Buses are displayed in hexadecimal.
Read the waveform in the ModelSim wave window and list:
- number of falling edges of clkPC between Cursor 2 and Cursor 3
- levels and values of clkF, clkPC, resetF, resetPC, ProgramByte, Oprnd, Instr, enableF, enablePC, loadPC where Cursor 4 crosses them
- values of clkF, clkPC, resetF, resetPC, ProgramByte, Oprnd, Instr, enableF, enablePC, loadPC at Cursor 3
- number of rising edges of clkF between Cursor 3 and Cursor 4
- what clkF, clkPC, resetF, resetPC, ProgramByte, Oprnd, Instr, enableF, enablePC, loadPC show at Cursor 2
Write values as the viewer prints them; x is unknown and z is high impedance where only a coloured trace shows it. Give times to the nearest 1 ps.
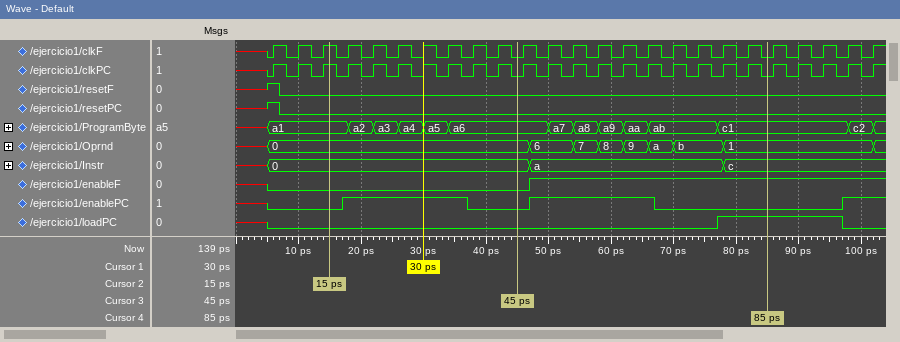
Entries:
8
clkF=0, clkPC=0, resetF=0, resetPC=0, ProgramByte=c1, Oprnd=1, Instr=c, enableF=1, enablePC=0, loadPC=1
clkF=0, clkPC=0, resetF=0, resetPC=0, ProgramByte=a6, Oprnd=0, Instr=0, enableF=0, enablePC=0, loadPC=0
10
clkF=1, clkPC=1, resetF=0, resetPC=0, ProgramByte=a1, Oprnd=0, Instr=0, enableF=0, enablePC=0, loadPC=0
